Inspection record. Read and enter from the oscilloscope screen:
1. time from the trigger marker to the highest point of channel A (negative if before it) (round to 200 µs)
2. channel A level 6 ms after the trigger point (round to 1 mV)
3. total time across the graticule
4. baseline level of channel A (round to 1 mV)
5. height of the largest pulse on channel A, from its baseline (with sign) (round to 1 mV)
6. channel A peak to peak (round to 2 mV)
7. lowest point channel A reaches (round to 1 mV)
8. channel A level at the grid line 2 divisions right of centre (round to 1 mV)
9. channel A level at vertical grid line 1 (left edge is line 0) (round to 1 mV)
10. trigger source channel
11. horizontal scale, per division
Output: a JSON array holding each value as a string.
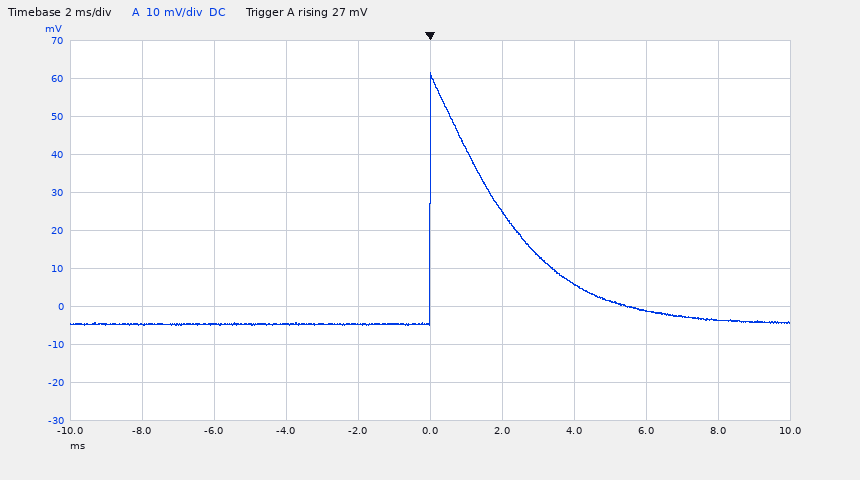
["0.0 ms", "-1 mV", "20 ms", "-5 mV", "+66 mV", "66 mV", "-5 mV", "6 mV", "-5 mV", "channel A", "2 ms"]
